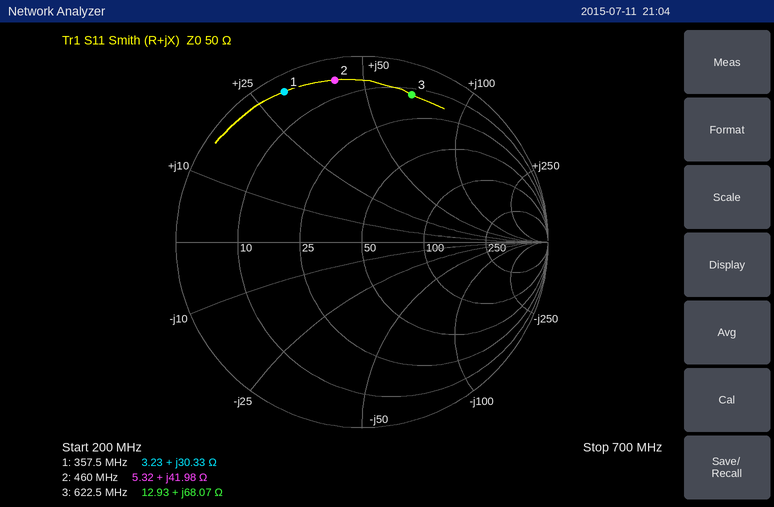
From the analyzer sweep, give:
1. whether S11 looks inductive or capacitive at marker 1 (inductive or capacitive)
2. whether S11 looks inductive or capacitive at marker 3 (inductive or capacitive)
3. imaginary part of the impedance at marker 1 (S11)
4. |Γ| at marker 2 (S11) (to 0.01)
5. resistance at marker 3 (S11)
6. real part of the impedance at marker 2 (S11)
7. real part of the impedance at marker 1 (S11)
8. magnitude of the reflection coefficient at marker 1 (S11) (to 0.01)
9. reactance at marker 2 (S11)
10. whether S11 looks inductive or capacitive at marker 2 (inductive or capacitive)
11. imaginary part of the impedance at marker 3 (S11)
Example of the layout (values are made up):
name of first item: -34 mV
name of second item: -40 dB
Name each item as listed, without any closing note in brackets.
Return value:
whether S11 looks inductive or capacitive at marker 1: inductive
whether S11 looks inductive or capacitive at marker 3: inductive
imaginary part of the impedance at marker 1: +30.33 Ω
|Γ| at marker 2 (S11): 0.88
resistance at marker 3: 12.93 Ω
real part of the impedance at marker 2: 5.32 Ω
real part of the impedance at marker 1: 3.23 Ω
magnitude of the reflection coefficient at marker 1 (S11): 0.91
reactance at marker 2: +41.98 Ω
whether S11 looks inductive or capacitive at marker 2: inductive
imaginary part of the impedance at marker 3: +68.07 Ω
